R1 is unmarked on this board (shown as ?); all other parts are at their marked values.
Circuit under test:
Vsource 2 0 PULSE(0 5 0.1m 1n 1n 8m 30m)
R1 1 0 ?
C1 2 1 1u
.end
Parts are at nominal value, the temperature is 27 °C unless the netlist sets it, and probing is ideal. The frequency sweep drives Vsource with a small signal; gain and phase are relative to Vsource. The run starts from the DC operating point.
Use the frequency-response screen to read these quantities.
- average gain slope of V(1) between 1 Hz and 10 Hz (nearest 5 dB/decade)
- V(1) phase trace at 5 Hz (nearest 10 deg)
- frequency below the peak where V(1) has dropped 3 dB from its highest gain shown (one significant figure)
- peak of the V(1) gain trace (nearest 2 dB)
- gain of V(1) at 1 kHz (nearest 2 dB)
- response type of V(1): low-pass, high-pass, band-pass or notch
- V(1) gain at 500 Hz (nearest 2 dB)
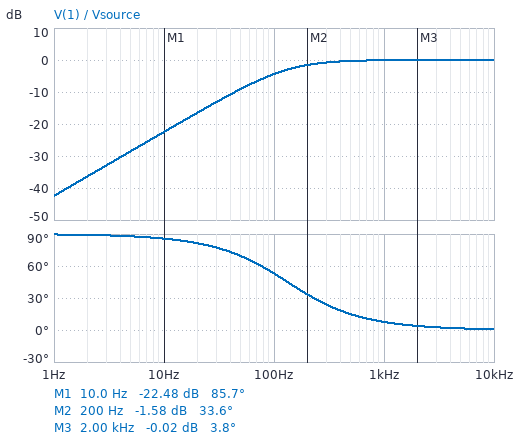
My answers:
20 dB/decade
90 deg
100 Hz
0 dB
0 dB
high-pass
0 dB
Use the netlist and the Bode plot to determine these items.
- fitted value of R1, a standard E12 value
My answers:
1.2 kΩ
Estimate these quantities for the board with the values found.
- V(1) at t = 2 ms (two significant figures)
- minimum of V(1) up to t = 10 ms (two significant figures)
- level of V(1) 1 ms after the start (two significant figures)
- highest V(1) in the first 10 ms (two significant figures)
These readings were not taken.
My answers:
1.0 V
-5.0 V
2.4 V
5.0 V
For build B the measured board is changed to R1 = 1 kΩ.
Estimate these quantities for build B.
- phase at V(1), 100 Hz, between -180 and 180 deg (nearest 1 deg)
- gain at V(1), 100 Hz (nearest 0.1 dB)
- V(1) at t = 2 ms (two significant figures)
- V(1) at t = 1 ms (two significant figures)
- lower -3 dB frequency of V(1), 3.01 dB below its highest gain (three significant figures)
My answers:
58 deg
-5.5 dB
750 mV
2.0 V
159 Hz
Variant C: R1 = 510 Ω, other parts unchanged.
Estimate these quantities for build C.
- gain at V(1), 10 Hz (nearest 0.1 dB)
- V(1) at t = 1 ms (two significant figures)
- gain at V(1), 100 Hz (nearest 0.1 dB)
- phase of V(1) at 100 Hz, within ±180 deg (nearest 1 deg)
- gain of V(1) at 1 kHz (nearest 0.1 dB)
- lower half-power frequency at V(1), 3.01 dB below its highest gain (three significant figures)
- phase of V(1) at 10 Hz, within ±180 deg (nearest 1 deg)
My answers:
-29.9 dB
860 mV
-10.3 dB
72 deg
-0.4 dB
312 Hz
88 deg
